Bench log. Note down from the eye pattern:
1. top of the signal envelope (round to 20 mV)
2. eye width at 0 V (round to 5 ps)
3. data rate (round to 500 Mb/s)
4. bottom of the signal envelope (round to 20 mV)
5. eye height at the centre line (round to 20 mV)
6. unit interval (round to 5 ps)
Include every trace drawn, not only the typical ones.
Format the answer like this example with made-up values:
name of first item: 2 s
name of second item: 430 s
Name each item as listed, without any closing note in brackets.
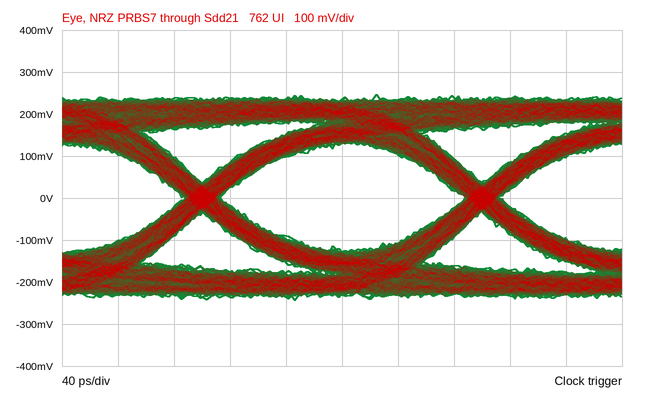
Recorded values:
top of the signal envelope: 240 mV
eye width at 0 V: 175 ps
data rate: 5.0 Gb/s
bottom of the signal envelope: -240 mV
eye height at the centre line: 260 mV
unit interval: 200 ps
